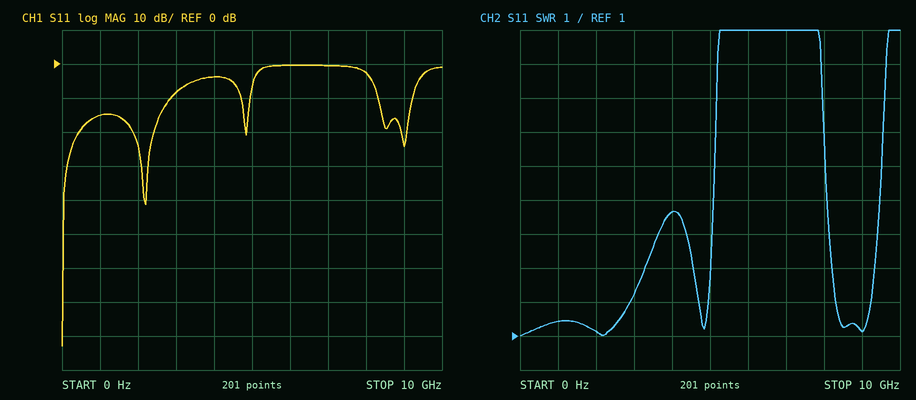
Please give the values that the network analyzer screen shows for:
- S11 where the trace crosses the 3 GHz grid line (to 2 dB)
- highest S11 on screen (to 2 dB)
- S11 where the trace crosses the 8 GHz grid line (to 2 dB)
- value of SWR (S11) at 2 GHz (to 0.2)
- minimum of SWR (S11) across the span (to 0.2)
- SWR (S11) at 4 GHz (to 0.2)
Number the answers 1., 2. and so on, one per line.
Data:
1. -8 dB
2. 0 dB
3. -2 dB
4. 1.2
5. 1.0
6. 4.6
